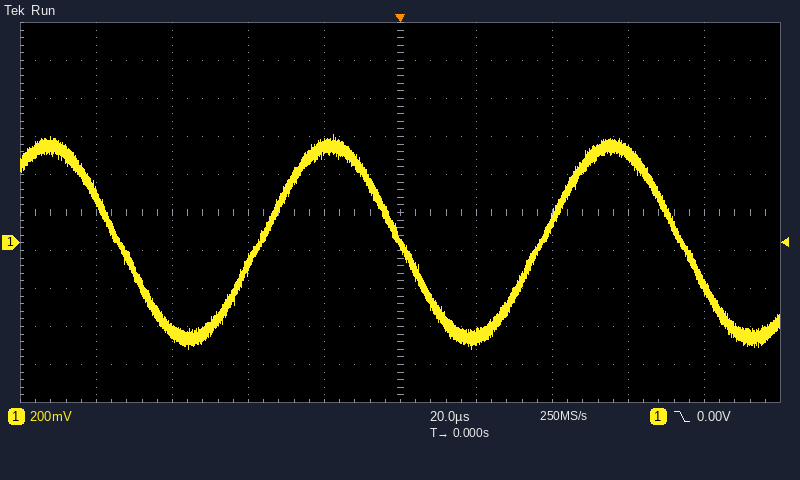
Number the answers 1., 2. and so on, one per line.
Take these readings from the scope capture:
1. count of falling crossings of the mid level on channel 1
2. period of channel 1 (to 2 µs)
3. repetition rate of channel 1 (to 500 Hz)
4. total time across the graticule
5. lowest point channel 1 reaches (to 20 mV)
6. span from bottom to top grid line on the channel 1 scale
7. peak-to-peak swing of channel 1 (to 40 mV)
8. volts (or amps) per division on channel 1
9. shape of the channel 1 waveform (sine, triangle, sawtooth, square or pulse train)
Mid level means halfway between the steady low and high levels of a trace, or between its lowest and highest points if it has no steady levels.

1. 3
2. 74 µs
3. 13.5 kHz
4. 200 µs
5. -560 mV
6. 2 V
7. 1.12 V
8. 200 mV
9. sine
